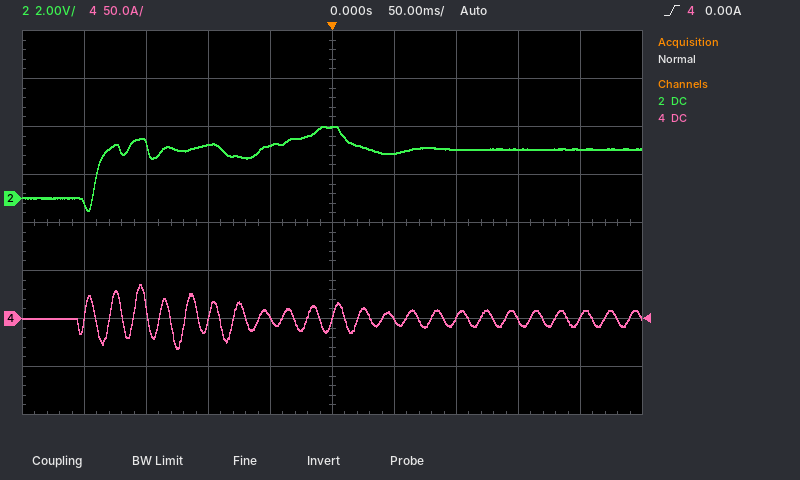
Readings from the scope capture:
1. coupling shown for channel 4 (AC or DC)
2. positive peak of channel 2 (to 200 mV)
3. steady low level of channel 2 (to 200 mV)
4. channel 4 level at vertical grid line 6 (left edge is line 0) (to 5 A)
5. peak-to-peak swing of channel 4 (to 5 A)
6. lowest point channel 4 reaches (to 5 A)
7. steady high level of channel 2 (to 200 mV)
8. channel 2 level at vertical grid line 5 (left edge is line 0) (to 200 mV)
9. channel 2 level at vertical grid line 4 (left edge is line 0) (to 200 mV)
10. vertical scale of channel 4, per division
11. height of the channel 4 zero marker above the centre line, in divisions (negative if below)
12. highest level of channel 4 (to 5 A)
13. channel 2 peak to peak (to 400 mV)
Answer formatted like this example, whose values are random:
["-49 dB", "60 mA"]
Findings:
["DC", "3.0 V", "0.0 V", "0 A", "65 A", "-30 A", "2.0 V", "3.0 V", "2.2 V", "50 A", "-2.0 div", "35 A", "3.6 V"]
